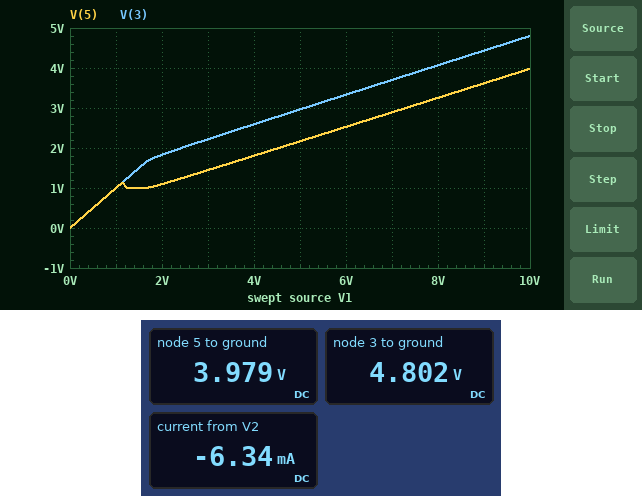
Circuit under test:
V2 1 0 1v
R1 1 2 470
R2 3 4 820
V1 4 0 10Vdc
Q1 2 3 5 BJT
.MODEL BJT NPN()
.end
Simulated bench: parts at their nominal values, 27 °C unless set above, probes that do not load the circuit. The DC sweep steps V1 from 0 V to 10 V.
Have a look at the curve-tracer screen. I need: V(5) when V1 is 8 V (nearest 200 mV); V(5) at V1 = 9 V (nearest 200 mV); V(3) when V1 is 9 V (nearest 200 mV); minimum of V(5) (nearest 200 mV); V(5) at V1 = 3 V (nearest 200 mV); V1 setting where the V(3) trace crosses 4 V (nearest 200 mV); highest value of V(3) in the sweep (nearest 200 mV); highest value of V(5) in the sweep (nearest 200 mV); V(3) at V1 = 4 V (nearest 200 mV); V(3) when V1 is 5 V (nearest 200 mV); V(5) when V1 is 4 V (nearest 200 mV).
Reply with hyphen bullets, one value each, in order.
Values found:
- 3.2 V
- 3.6 V
- 4.4 V
- 0 V
- 1.4 V
- 7.8 V
- 4.8 V
- 4.0 V
- 2.6 V
- 3.0 V
- 1.8 V
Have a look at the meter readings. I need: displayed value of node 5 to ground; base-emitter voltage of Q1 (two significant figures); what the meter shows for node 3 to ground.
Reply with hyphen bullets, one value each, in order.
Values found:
- 3.979 V
- 820 mV
- 4.802 V
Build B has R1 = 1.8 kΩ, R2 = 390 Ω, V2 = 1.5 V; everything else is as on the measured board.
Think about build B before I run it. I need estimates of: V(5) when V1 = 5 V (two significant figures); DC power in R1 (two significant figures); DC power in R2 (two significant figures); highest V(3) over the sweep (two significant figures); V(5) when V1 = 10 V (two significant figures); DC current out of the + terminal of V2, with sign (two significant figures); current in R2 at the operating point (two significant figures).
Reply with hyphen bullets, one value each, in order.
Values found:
- 3.7 V
- 22 mW
- 4.8 mW
- 8.6 V
- 7.8 V
- -3.5 mA
- 3.5 mA
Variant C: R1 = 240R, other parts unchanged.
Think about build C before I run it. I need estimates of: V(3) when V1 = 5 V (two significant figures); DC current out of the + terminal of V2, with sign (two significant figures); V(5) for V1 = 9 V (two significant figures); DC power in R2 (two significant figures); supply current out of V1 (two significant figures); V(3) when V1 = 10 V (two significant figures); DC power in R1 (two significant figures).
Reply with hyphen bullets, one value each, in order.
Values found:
- 2.5 V
- -7.7 mA
- 2.6 V
- 49 mW
- 7.7 mA
- 3.7 V
- 14 mW
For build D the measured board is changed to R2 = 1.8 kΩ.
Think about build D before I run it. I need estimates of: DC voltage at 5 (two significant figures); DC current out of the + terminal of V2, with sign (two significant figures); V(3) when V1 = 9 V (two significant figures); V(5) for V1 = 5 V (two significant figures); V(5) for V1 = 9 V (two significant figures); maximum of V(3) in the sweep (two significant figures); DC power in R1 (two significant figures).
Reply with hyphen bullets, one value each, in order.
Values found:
- 2.7 V
- -3.6 mA
- 3.3 V
- 1.7 V
- 2.5 V
- 3.5 V
- 6.1 mW
